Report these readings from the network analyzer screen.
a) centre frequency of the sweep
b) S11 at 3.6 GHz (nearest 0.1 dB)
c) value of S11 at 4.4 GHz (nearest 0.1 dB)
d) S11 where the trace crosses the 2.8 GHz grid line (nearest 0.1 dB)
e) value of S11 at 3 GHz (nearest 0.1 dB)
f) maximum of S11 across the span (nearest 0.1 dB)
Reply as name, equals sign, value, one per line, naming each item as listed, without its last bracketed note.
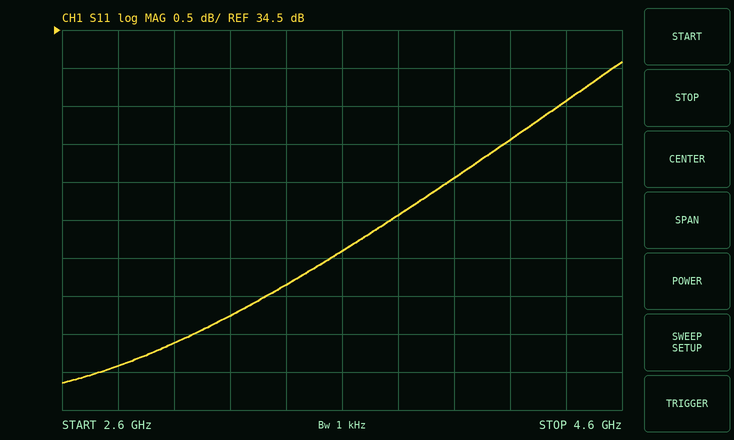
centre frequency of the sweep = 3.6 GHz
S11 at 3.6 GHz = 31.6 dB
value of S11 at 4.4 GHz = 33.6 dB
S11 where the trace crosses the 2.8 GHz grid line = 30.1 dB
value of S11 at 3 GHz = 30.4 dB
maximum of S11 across the span = 34.1 dB
